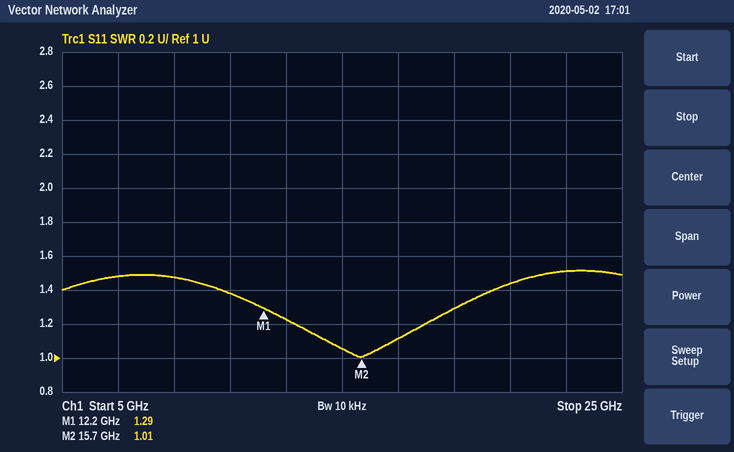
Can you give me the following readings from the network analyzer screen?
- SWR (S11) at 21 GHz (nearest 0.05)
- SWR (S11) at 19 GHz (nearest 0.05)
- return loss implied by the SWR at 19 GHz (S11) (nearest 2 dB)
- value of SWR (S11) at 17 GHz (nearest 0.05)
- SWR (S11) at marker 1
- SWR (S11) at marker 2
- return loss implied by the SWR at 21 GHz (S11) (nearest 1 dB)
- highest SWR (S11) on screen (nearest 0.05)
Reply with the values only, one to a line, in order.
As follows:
1.45
1.30
18 dB
1.10
1.29
1.01
15 dB
1.50
